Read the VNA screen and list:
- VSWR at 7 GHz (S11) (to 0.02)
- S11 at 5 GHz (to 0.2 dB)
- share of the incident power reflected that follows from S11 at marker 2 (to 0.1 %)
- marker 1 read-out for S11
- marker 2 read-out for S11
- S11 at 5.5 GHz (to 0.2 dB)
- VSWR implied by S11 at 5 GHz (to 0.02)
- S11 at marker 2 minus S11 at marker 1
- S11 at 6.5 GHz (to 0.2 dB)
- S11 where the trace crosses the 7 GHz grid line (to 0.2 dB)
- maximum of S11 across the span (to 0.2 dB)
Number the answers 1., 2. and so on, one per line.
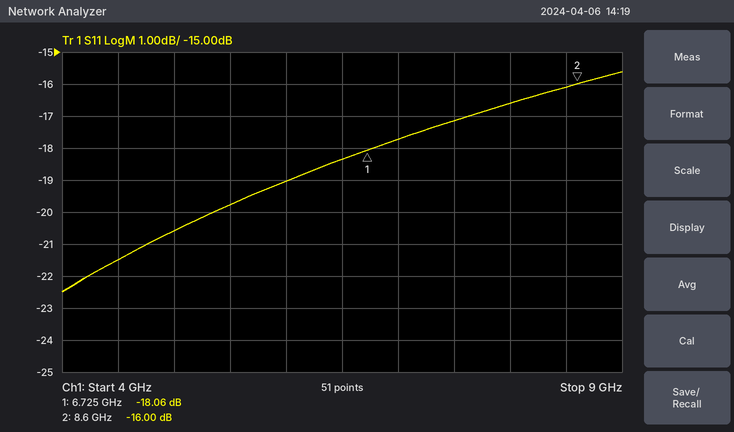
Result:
1. 1.30
2. -20.6 dB
3. 2.5 %
4. -18.06 dB
5. -16.00 dB
6. -19.8 dB
7. 1.20
8. 2.06 dB
9. -18.4 dB
10. -17.8 dB
11. -15.6 dB
